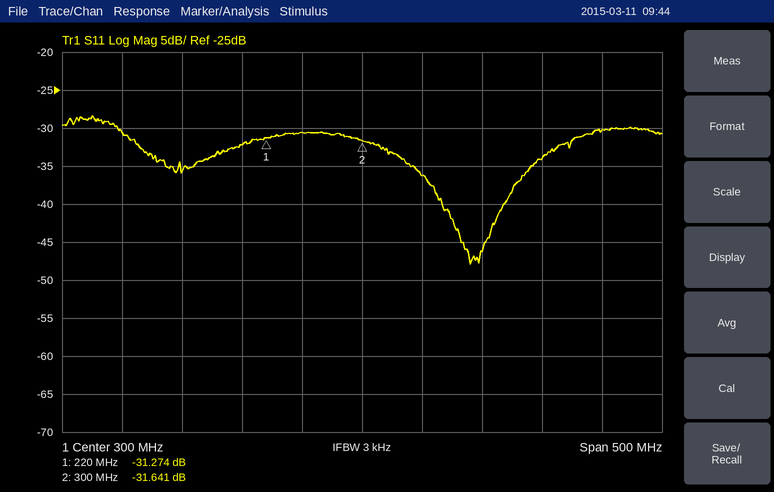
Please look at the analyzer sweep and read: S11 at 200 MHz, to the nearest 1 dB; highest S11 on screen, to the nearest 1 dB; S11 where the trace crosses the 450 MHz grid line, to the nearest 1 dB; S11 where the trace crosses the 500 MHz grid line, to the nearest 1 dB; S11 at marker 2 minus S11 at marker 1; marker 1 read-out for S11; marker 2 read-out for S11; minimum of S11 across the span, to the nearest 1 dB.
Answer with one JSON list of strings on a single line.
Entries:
["-32 dB", "-28 dB", "-34 dB", "-30 dB", "-0.367 dB", "-31.274 dB", "-31.641 dB", "-48 dB"]
